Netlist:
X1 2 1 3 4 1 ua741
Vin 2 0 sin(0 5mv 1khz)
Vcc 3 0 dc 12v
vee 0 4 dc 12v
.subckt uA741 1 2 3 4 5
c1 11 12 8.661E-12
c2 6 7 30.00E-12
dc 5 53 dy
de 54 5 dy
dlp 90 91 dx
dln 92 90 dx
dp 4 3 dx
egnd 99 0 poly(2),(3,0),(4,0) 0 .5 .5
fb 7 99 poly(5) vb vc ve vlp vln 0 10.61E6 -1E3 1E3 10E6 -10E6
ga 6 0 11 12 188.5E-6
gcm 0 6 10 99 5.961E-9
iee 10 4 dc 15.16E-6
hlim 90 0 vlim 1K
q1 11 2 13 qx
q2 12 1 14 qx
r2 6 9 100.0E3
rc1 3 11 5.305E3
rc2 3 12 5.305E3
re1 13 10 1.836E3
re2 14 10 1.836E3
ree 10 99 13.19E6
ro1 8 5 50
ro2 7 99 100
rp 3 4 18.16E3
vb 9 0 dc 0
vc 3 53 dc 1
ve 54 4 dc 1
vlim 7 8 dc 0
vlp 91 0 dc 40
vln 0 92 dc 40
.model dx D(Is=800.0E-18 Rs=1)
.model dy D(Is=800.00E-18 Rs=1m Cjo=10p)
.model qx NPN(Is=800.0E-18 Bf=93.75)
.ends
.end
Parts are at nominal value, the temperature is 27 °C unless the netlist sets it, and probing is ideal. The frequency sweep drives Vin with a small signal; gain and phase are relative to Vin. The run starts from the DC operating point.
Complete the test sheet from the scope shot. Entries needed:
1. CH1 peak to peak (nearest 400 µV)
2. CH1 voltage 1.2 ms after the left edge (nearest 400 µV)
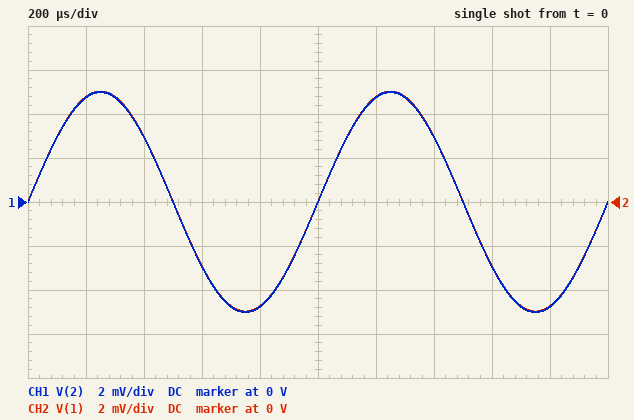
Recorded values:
10.0 mV
4.8 mV
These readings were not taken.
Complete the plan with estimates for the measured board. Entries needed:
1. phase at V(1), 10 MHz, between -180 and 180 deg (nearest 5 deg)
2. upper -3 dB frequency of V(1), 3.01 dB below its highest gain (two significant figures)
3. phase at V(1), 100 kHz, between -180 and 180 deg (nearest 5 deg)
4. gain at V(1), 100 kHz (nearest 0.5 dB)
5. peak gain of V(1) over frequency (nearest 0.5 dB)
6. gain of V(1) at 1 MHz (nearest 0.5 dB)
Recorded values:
-170 deg
1.4 MHz
-5 deg
0 dB
0 dB
-0.5 dB
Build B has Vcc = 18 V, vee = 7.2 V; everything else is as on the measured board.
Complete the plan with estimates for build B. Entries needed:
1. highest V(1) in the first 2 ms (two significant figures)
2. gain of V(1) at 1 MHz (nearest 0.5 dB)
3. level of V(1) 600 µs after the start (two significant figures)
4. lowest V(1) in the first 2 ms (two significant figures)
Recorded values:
5.2 mV
-1.0 dB
-2.7 mV
-4.8 mV
